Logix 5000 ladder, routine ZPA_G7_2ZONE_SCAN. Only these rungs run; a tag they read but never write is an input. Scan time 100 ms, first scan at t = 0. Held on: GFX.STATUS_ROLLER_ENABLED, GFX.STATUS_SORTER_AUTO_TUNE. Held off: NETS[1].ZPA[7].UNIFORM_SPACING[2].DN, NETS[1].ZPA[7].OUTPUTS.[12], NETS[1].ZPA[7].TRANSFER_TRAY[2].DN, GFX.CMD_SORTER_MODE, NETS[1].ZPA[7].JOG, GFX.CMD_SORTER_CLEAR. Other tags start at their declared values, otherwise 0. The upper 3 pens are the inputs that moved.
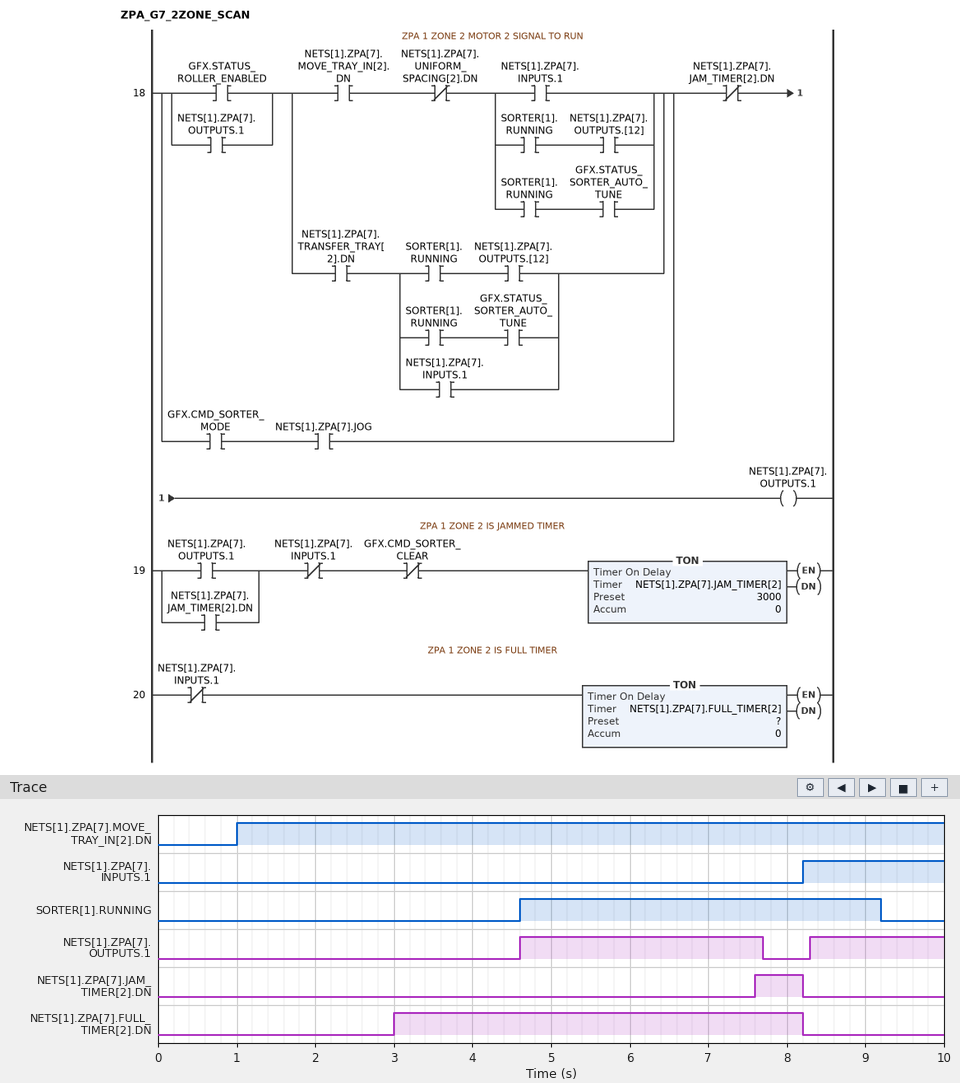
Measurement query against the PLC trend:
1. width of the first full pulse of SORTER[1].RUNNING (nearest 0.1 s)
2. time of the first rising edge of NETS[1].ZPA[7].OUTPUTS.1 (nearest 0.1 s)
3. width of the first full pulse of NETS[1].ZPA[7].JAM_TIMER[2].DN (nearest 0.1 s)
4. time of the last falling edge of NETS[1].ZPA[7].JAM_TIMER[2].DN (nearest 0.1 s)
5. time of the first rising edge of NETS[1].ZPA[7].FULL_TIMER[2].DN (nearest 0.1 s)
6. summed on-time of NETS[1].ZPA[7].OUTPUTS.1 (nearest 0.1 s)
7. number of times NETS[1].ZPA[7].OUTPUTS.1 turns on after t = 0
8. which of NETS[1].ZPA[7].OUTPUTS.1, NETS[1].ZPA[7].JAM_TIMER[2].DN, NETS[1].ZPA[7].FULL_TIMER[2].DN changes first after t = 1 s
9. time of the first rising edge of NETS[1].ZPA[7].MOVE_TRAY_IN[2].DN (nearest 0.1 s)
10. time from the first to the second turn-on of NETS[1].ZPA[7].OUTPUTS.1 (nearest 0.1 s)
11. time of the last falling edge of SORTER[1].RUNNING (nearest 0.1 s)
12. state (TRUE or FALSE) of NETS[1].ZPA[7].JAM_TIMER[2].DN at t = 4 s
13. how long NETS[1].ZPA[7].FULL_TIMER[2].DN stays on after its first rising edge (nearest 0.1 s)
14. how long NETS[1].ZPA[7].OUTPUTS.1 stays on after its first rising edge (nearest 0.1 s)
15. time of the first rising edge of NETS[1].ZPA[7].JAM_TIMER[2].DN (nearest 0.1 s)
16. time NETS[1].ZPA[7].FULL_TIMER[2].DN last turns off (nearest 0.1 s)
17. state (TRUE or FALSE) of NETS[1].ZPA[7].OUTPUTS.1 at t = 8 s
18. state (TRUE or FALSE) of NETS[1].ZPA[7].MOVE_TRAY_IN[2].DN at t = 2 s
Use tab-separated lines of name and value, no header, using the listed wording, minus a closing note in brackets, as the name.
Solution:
width of the first full pulse of SORTER[1].RUNNING	4.6 s
time of the first rising edge of NETS[1].ZPA[7].OUTPUTS.1	4.6 s
width of the first full pulse of NETS[1].ZPA[7].JAM_TIMER[2].DN	0.6 s
time of the last falling edge of NETS[1].ZPA[7].JAM_TIMER[2].DN	8.2 s
time of the first rising edge of NETS[1].ZPA[7].FULL_TIMER[2].DN	3.0 s
summed on-time of NETS[1].ZPA[7].OUTPUTS.1	4.8 s
number of times NETS[1].ZPA[7].OUTPUTS.1 turns on after t = 0	2
which of NETS[1].ZPA[7].OUTPUTS.1, NETS[1].ZPA[7].JAM_TIMER[2].DN, NETS[1].ZPA[7].FULL_TIMER[2].DN changes first after t = 1 s	NETS[1].ZPA[7].FULL_TIMER[2].DN
time of the first rising edge of NETS[1].ZPA[7].MOVE_TRAY_IN[2].DN	1.0 s
time from the first to the second turn-on of NETS[1].ZPA[7].OUTPUTS.1	3.7 s
time of the last falling edge of SORTER[1].RUNNING	9.2 s
state (TRUE or FALSE) of NETS[1].ZPA[7].JAM_TIMER[2].DN at t = 4 s	FALSE
how long NETS[1].ZPA[7].FULL_TIMER[2].DN stays on after its first rising edge	5.2 s
how long NETS[1].ZPA[7].OUTPUTS.1 stays on after its first rising edge	3.1 s
time of the first rising edge of NETS[1].ZPA[7].JAM_TIMER[2].DN	7.6 s
time NETS[1].ZPA[7].FULL_TIMER[2].DN last turns off	8.2 s
state (TRUE or FALSE) of NETS[1].ZPA[7].OUTPUTS.1 at t = 8 s	FALSE
state (TRUE or FALSE) of NETS[1].ZPA[7].MOVE_TRAY_IN[2].DN at t = 2 s	TRUE
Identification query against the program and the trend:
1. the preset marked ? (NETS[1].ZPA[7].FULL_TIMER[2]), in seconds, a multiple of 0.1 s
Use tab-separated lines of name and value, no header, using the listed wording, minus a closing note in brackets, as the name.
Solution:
the preset marked ? (NETS[1].ZPA[7].FULL_TIMER[2]), in seconds, a multiple of 0.1 s	3.0 s
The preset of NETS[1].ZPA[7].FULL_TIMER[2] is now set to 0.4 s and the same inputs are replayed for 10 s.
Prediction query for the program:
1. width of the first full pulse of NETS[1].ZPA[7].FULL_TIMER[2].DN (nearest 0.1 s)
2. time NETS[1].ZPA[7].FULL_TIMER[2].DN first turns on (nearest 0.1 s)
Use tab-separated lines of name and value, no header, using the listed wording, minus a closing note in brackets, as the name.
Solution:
width of the first full pulse of NETS[1].ZPA[7].FULL_TIMER[2].DN	7.8 s
time NETS[1].ZPA[7].FULL_TIMER[2].DN first turns on	0.4 s
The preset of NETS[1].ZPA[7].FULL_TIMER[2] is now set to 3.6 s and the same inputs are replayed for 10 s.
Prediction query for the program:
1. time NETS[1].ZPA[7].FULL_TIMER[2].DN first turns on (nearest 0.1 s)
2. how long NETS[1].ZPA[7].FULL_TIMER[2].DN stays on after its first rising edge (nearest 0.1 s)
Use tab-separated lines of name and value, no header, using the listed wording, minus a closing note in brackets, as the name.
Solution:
time NETS[1].ZPA[7].FULL_TIMER[2].DN first turns on	3.6 s
how long NETS[1].ZPA[7].FULL_TIMER[2].DN stays on after its first rising edge	4.6 s
